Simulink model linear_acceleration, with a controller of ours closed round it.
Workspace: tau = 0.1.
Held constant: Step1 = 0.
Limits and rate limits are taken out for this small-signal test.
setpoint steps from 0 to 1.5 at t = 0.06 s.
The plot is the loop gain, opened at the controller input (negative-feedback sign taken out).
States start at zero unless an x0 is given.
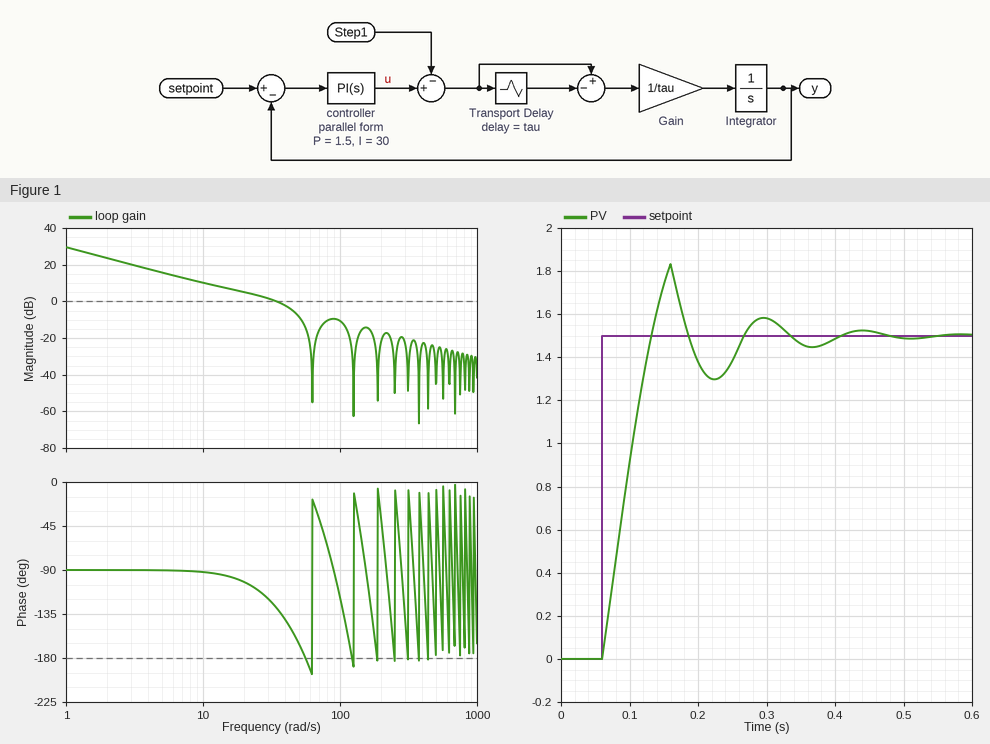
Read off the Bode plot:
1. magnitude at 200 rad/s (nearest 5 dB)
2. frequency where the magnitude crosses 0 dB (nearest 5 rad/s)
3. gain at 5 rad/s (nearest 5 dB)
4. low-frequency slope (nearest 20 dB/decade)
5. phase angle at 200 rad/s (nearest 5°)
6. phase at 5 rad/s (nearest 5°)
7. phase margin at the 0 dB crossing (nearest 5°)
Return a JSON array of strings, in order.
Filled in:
["-20 dB", "35 rad/s", "15 dB", "-20 dB/decade", "-40°", "-90°", "50°"]
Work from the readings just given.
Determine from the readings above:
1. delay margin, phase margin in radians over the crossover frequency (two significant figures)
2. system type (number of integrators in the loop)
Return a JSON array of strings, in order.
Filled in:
["0.025 s", "1"]
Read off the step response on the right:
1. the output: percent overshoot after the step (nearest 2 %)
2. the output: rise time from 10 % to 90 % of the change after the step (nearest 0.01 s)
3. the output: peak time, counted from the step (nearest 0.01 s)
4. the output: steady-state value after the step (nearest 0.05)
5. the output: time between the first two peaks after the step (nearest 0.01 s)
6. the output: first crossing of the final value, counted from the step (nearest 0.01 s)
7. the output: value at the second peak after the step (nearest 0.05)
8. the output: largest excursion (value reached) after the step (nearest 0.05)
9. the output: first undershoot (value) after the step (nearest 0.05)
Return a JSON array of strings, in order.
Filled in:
["22 %", "0.06 s", "0.10 s", "1.50", "0.14 s", "0.07 s", "1.60", "1.85", "1.30"]
